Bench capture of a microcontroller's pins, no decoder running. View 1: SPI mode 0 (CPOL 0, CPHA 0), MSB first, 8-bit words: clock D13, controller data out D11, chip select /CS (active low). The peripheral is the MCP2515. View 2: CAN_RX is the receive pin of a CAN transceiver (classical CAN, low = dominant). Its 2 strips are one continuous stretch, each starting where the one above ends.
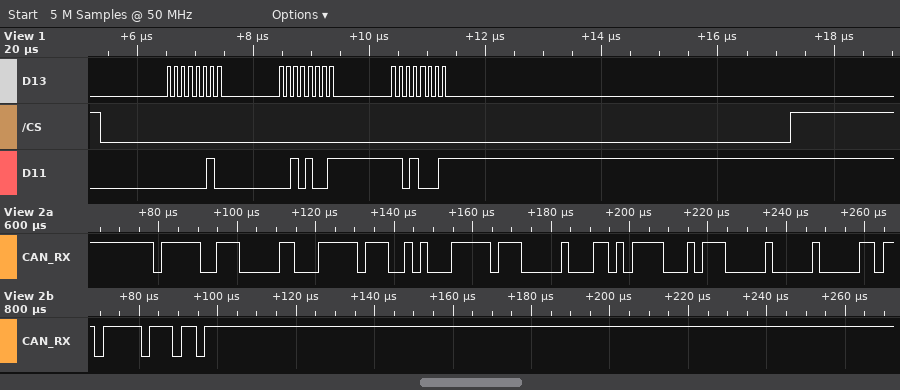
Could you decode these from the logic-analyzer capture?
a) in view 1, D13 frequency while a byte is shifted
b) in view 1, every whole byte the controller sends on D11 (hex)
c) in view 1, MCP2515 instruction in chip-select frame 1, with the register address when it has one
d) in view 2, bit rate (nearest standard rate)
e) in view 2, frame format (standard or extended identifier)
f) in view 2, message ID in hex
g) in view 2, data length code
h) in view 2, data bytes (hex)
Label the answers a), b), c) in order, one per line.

a) 8 MHz
b) 02 29 D1
c) WRITE 0x29
d) 500 kbit/s
e) standard
f) 0x7DC
g) 8
h) FF 28 FF 00 D7 8B 80 00
